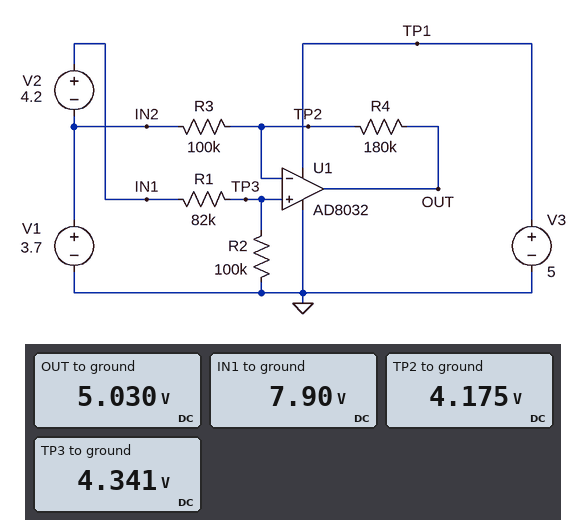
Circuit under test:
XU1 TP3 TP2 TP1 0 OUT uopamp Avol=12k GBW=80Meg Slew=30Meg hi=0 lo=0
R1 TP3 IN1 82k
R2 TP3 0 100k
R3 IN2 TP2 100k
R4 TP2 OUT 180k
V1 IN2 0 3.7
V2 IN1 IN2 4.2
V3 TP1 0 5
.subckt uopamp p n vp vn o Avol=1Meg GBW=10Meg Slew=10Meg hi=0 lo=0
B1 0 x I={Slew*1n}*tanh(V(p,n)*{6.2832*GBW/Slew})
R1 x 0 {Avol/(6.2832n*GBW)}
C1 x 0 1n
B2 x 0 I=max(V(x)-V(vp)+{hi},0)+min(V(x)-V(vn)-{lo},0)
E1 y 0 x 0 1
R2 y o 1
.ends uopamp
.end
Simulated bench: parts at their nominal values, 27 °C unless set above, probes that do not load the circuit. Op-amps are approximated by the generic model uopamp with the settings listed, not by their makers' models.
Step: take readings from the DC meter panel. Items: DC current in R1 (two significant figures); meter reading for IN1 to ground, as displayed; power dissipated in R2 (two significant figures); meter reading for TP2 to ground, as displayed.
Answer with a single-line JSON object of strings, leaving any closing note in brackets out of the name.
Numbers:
{"DC current in R1": "43 µA", "meter reading for IN1 to ground, as displayed": "7.90 V", "power dissipated in R2": "190 µW", "meter reading for TP2 to ground, as displayed": "4.175 V"}
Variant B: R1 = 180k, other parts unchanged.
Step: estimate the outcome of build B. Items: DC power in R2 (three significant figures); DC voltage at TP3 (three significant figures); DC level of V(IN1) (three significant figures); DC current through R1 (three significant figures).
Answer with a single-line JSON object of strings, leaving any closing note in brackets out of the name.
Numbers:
{"DC power in R2": "79.6 µW", "DC voltage at TP3": "2.82 V", "DC level of V(IN1)": "7.90 V", "DC current through R1": "28.2 µA"}
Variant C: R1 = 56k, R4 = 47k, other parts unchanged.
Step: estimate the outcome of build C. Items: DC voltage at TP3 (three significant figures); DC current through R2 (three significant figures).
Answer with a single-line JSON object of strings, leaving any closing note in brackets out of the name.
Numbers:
{"DC voltage at TP3": "5.06 V", "DC current through R2": "50.6 µA"}
